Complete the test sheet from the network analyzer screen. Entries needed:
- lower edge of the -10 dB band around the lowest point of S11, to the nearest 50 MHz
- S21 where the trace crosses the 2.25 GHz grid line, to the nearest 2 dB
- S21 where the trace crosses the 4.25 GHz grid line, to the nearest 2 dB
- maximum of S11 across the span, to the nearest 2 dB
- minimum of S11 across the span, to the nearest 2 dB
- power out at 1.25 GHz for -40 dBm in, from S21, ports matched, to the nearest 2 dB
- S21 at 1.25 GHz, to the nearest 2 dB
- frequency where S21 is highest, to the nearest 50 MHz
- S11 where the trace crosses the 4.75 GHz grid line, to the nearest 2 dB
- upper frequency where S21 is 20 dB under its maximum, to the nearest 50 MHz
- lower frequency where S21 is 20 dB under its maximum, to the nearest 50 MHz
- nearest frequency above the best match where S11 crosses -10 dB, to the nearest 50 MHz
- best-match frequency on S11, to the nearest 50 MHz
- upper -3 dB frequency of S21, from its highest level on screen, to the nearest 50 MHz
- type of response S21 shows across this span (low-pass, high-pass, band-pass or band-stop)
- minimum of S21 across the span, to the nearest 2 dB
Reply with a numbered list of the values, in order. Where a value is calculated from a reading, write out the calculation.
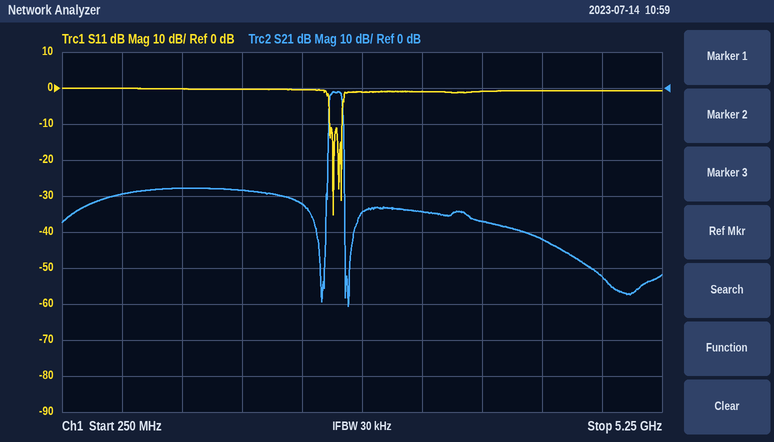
1. 2.50 GHz
2. -32 dB
3. -42 dB
4. 0 dB
5. -36 dB
6. -40 dBm + (-28 dB) = -68 dBm
7. -28 dB
8. 2.50 GHz
9. 0 dB
10. 2.60 GHz
11. 2.45 GHz
12. 2.60 GHz
13. 2.50 GHz
14. 2.60 GHz
15. band-pass
16. -60 dB
